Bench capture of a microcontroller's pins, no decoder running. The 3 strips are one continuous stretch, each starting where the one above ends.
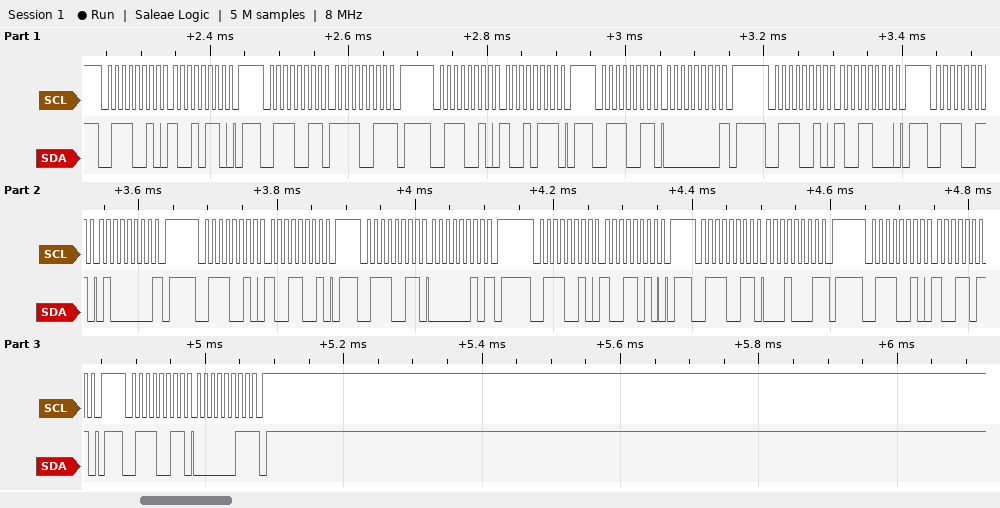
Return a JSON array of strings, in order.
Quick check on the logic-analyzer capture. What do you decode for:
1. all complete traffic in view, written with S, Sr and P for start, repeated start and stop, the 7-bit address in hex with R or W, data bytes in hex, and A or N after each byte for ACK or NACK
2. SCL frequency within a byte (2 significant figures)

["S 39W A 96 A P S 39R A F3 N P S 39W A 97 A P S 39R A 00 N P S 39W A 98 A P S 39R A 40 N P S 39W A 99 A P S 39R A 02 N P S 39W A 9A A P S 39R A 11 N P S 39W A 9B A P S 39R A 03 N P", "100 kHz"]
